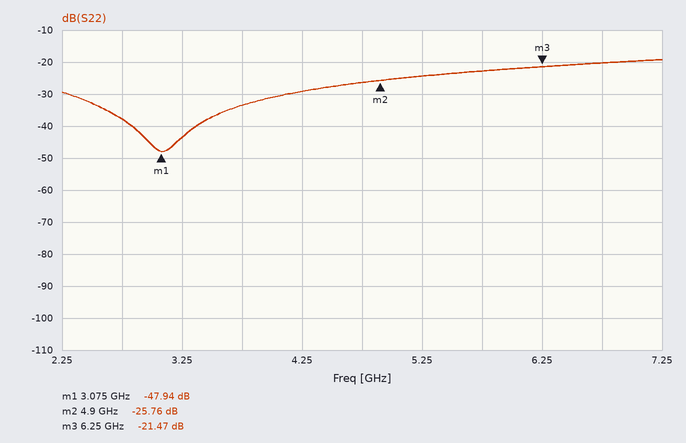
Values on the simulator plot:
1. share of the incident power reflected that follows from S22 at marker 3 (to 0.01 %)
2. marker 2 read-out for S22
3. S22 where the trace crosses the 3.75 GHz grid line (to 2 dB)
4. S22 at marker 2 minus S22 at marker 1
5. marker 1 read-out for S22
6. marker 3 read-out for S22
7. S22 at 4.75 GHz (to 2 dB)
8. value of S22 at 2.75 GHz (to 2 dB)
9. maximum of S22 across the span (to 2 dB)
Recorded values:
0.71 %
-25.76 dB
-34 dB
22.18 dB
-47.94 dB
-21.47 dB
-26 dB
-38 dB
-20 dB
